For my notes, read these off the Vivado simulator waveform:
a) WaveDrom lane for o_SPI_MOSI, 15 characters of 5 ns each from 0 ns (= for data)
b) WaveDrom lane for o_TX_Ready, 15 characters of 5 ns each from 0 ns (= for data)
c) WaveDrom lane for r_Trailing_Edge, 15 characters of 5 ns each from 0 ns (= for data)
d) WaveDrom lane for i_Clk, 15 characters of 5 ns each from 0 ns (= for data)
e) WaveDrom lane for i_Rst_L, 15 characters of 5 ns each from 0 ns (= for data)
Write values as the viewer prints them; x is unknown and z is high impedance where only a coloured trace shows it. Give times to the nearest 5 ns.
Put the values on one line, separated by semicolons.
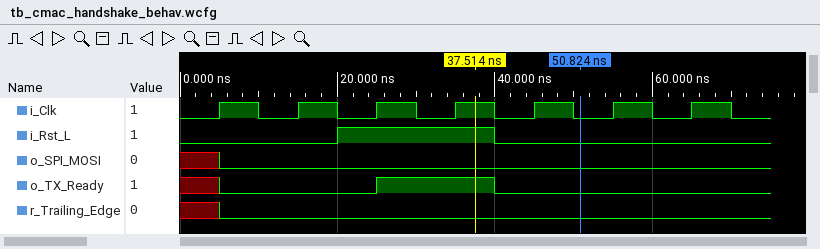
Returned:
{name: 'o_SPI_MOSI', wave: 'x0.............'}; {name: 'o_TX_Ready', wave: 'x0...1..0......'}; {name: 'r_Trailing_Edge', wave: 'x0.............'}; {name: 'i_Clk', wave: '010101010101010'}; {name: 'i_Rst_L', wave: '0...1...0......'}
